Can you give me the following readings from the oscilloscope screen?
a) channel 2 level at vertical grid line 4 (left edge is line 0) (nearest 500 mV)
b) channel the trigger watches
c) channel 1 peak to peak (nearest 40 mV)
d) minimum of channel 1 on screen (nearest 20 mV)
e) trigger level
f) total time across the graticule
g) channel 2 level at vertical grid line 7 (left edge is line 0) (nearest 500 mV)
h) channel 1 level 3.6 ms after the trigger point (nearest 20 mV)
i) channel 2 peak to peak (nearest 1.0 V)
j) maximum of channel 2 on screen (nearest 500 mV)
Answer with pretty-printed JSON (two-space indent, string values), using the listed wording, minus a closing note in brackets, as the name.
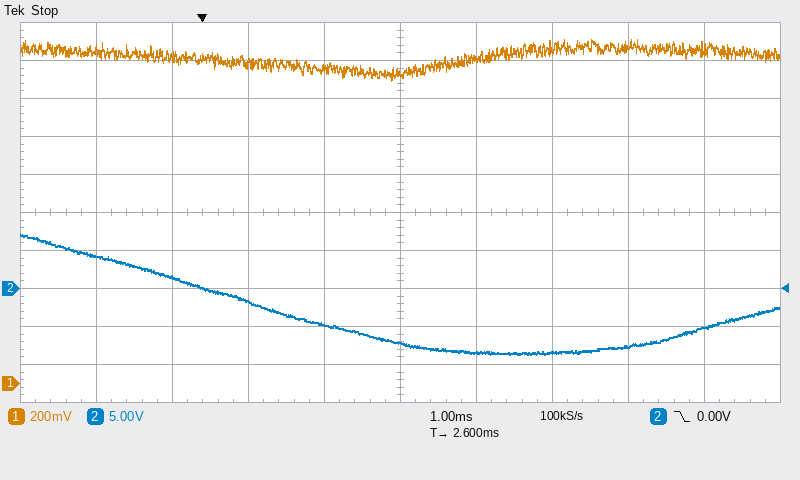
{
  "channel 2 level at vertical grid line 4 (left edge is line 0)": "-4.5 V",
  "channel the trigger watches": "channel 2",
  "channel 1 peak to peak": "200 mV",
  "minimum of channel 1 on screen": "1.60 V",
  "trigger level": "0.00 V",
  "total time across the graticule": "10 ms",
  "channel 2 level at vertical grid line 7 (left edge is line 0)": "-8.5 V",
  "channel 1 level 3.6 ms after the trigger point": "1.70 V",
  "channel 2 peak to peak": "16.0 V",
  "maximum of channel 2 on screen": "7.0 V"
}
